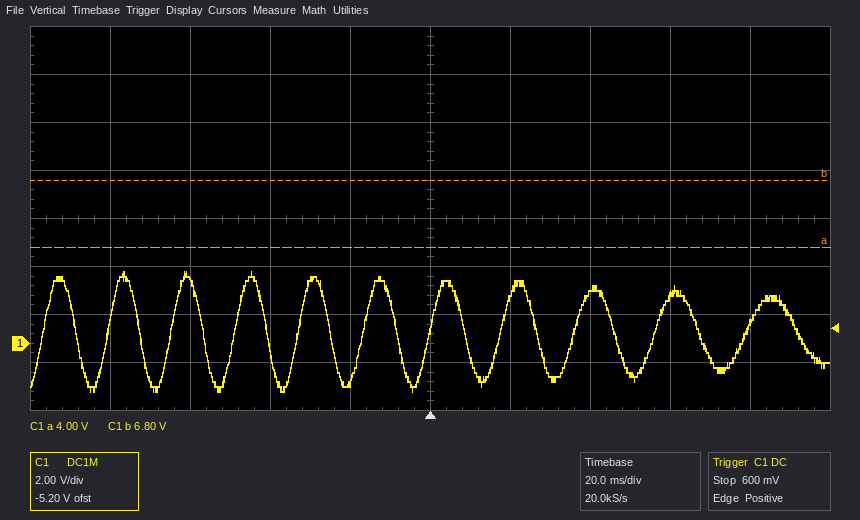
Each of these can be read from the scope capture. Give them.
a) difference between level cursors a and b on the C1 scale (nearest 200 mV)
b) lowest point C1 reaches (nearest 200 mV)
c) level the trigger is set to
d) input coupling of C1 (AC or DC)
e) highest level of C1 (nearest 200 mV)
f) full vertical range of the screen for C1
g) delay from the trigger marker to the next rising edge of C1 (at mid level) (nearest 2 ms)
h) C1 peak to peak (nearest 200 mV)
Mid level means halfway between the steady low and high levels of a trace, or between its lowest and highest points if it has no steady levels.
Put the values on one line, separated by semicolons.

2.8 V; -2.0 V; 600 mV; DC; 3.0 V; 16 V; 18 ms; 5.0 V
